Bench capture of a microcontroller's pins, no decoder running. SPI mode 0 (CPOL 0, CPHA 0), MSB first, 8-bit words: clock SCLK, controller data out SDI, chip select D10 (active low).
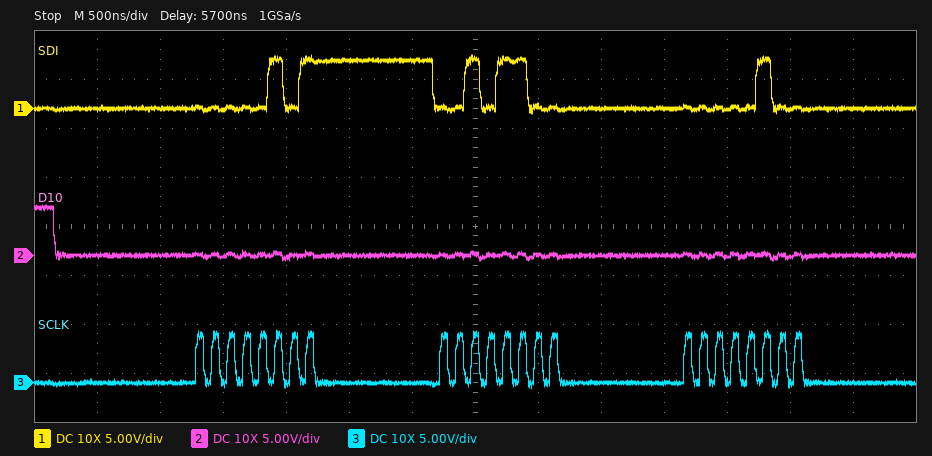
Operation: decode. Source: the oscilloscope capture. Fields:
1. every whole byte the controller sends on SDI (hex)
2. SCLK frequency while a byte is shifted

0x05 0x2C 0x04
8 MHz
